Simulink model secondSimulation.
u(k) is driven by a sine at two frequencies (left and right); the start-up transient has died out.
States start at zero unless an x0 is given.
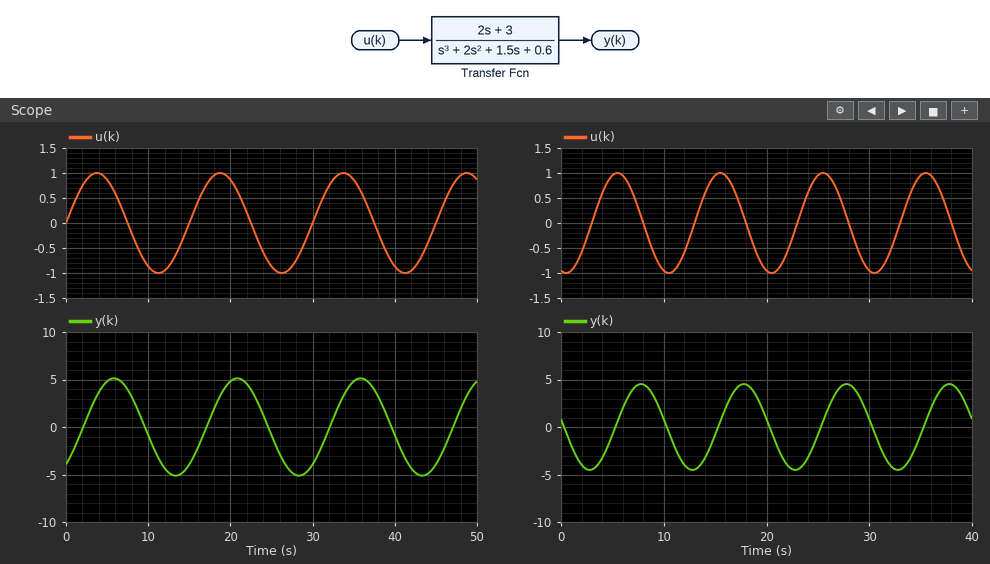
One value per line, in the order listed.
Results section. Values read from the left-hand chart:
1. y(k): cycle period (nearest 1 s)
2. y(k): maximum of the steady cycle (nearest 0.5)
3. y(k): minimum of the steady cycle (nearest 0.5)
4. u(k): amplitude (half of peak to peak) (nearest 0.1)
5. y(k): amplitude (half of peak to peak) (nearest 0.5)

15 s
5.0
-5.0
1.0
5.0
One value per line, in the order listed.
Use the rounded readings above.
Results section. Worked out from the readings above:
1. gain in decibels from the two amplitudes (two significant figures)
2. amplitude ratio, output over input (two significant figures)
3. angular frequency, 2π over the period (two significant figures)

14 dB
5.0
0.42 rad/s
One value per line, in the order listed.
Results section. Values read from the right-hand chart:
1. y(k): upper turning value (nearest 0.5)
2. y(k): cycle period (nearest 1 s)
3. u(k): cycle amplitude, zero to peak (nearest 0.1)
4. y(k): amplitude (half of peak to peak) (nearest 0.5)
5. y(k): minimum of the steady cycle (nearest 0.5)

4.5
10 s
1.0
4.5
-4.5
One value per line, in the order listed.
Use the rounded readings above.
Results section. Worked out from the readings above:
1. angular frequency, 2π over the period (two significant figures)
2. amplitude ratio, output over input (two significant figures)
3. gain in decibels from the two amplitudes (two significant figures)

0.63 rad/s
4.5
13 dB
